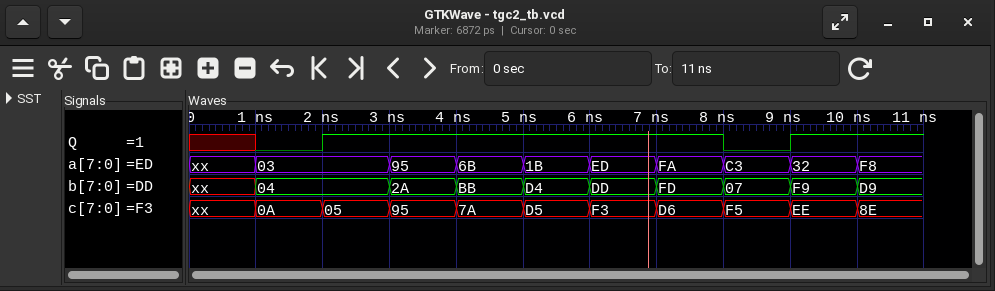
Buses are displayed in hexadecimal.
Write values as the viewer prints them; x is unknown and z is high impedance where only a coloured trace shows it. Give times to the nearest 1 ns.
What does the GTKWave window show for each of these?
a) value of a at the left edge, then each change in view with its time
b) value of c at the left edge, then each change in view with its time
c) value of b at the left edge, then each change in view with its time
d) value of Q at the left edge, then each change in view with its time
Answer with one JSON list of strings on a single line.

["xx, 03 at 1 ns, 95 at 3 ns, 6B at 4 ns, 1B at 5 ns, ED at 6 ns, FA at 7 ns, C3 at 8 ns, 32 at 9 ns, F8 at 10 ns", "xx, 0A at 1 ns, 05 at 2 ns, 95 at 3 ns, 7A at 4 ns, D5 at 5 ns, F3 at 6 ns, D6 at 7 ns, F5 at 8 ns, EE at 9 ns, 8E at 10 ns", "xx, 04 at 1 ns, 2A at 3 ns, BB at 4 ns, D4 at 5 ns, DD at 6 ns, FD at 7 ns, 07 at 8 ns, F9 at 9 ns, D9 at 10 ns", "x, 0 at 1 ns, 1 at 2 ns, 0 at 8 ns, 1 at 9 ns"]
